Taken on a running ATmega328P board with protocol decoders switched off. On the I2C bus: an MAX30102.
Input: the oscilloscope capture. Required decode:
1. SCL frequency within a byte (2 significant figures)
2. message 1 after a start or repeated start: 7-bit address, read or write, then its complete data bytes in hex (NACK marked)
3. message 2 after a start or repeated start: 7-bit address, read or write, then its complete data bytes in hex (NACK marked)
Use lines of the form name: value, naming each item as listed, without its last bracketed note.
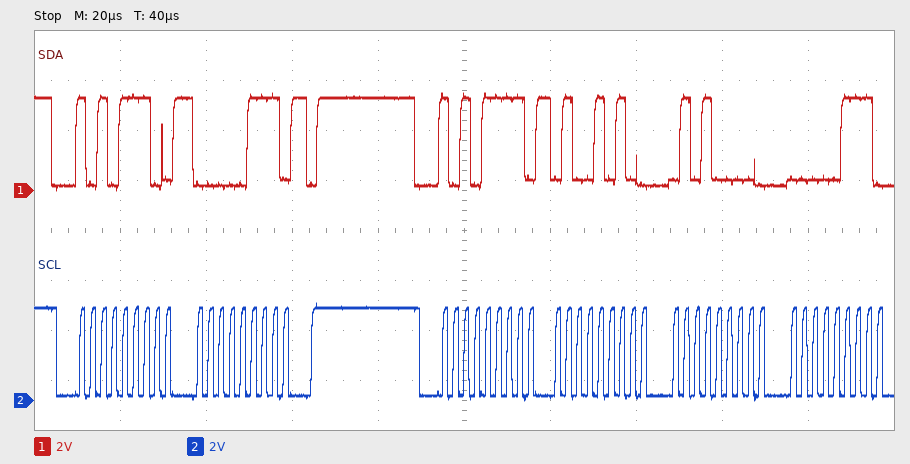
SCL frequency within a byte: 400 kHz
message 1 after a start or repeated start: 7-bit address, read or write, then its complete data bytes in hex: 0x57 write: 07
message 2 after a start or repeated start: 7-bit address, read or write, then its complete data bytes in hex: 0x57 read: 4A 50 07
